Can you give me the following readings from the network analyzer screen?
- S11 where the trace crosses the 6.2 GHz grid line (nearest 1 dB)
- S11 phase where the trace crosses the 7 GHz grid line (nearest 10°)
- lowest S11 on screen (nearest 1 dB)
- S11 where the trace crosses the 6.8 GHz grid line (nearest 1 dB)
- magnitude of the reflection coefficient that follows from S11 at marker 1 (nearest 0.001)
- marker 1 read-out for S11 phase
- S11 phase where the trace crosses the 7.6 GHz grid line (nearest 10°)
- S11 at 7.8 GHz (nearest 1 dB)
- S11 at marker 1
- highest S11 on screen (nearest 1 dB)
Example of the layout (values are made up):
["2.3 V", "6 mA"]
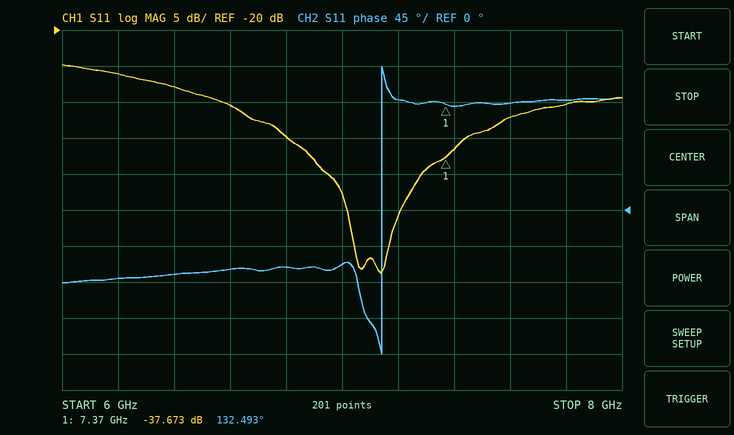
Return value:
["-26 dB", "-70°", "-54 dB", "-35 dB", "0.013", "132.493°", "130°", "-30 dB", "-37.673 dB", "-25 dB"]
